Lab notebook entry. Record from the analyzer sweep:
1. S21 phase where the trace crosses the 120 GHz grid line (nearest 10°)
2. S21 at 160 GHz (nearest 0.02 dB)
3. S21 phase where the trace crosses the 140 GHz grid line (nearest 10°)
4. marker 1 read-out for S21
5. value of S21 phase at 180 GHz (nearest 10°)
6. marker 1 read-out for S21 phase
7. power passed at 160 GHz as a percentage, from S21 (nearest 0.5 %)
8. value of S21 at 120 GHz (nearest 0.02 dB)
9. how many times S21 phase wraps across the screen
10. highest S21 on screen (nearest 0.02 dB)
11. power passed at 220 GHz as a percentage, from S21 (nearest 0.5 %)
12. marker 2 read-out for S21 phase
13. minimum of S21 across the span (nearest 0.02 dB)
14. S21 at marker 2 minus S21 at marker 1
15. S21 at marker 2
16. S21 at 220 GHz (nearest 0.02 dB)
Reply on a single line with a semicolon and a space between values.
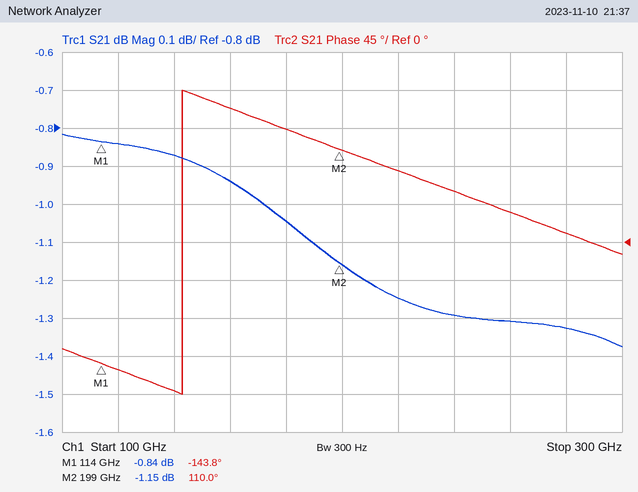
-150°; -0.94 dB; -180°; -0.84 dB; 130°; -143.8°; 80.5 %; -0.84 dB; 1; -0.82 dB; 75.0 %; 110.0°; -1.38 dB; -0.31 dB; -1.15 dB; -1.24 dB
